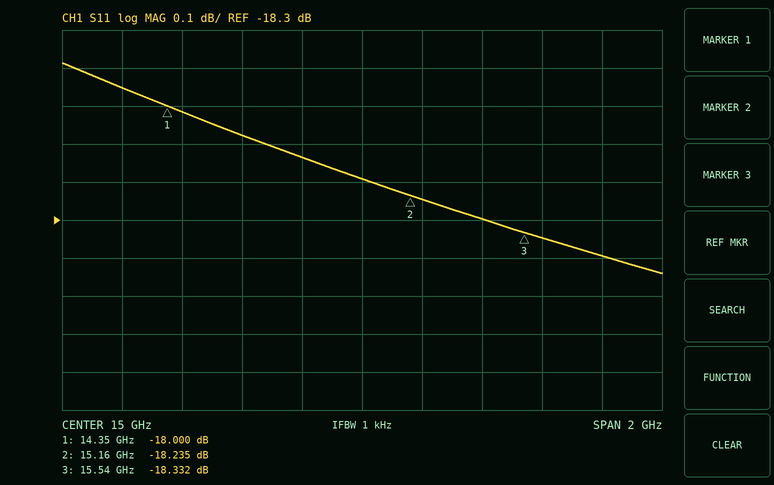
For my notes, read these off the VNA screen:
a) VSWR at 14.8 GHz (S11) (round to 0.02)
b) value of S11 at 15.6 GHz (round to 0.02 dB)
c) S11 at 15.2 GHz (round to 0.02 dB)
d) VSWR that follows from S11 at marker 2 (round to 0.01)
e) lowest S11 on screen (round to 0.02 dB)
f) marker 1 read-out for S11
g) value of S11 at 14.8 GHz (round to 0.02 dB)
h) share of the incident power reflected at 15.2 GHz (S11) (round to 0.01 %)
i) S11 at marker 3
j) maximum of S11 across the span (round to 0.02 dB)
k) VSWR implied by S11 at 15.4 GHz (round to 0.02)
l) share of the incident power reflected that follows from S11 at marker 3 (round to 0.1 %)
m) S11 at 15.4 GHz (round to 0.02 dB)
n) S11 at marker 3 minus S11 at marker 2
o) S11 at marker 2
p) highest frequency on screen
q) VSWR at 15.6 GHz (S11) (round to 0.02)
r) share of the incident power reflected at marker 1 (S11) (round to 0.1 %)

1.28
-18.34 dB
-18.24 dB
1.28
-18.44 dB
-18.000 dB
-18.14 dB
1.50 %
-18.332 dB
-17.88 dB
1.28
1.5 %
-18.30 dB
-0.097 dB
-18.235 dB
16 GHz
1.28
1.6 %
